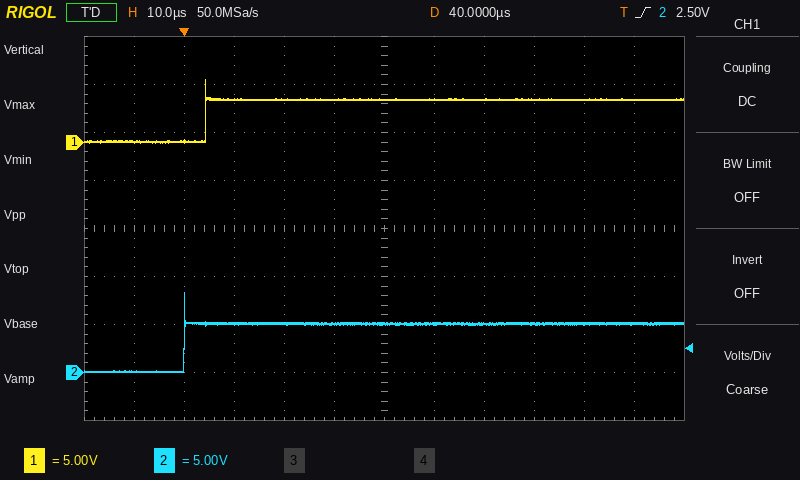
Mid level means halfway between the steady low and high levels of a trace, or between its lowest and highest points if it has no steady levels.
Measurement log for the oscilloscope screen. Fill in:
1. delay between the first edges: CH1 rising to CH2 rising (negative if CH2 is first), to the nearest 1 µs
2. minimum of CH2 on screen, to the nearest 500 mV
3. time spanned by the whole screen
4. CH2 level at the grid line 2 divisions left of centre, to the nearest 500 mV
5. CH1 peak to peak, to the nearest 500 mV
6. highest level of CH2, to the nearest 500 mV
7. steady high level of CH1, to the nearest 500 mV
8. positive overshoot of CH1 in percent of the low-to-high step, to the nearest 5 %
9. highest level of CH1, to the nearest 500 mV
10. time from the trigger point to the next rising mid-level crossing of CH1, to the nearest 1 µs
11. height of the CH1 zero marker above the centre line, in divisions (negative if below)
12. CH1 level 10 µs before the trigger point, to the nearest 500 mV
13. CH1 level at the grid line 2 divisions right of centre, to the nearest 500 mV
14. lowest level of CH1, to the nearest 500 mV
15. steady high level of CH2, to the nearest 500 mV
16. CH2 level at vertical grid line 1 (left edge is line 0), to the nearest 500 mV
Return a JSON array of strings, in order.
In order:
["-4 µs", "0.0 V", "120 µs", "5.0 V", "6.5 V", "8.5 V", "4.5 V", "50 %", "6.5 V", "4 µs", "+1.8 div", "0.0 V", "4.5 V", "0.0 V", "5.0 V", "0.0 V"]
